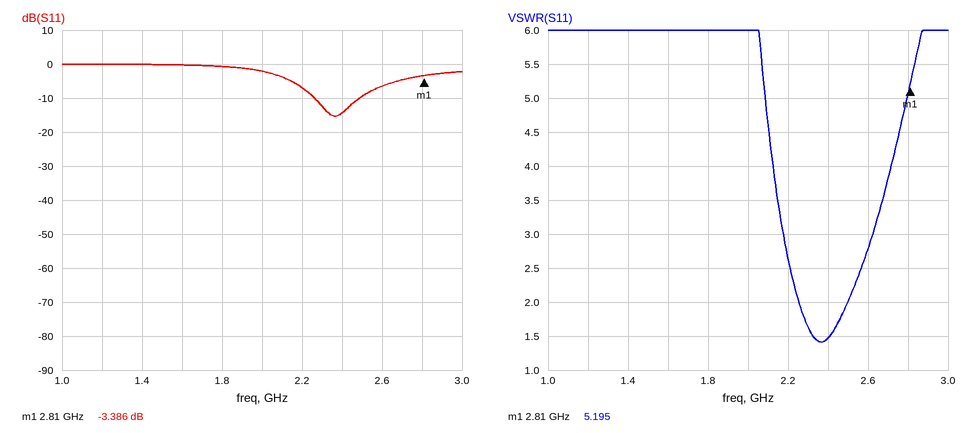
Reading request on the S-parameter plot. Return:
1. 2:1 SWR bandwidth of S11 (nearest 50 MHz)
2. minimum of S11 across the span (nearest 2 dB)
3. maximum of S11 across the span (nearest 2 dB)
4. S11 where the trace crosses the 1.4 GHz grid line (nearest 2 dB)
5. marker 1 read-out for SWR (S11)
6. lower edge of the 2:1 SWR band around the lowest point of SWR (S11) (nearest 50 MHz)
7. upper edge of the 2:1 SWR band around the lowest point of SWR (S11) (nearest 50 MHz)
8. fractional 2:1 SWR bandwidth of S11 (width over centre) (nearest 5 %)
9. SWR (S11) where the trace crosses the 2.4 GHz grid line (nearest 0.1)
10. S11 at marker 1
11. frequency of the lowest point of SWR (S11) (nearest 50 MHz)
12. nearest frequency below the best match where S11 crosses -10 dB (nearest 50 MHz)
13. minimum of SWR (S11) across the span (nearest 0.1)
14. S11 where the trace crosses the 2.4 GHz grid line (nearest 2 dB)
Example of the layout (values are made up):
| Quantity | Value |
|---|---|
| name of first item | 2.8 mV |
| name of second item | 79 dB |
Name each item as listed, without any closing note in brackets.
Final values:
| Quantity | Value |
|---|---|
| 2:1 SWR bandwidth of S11 | 250 MHz |
| minimum of S11 across the span | -16 dB |
| maximum of S11 across the span | 0 dB |
| S11 where the trace crosses the 1.4 GHz grid line | 0 dB |
| marker 1 read-out for SWR | 5.195 |
| lower edge of the 2:1 SWR band around the lowest point of SWR (S11) | 2.25 GHz |
| upper edge of the 2:1 SWR band around the lowest point of SWR (S11) | 2.50 GHz |
| fractional 2:1 SWR bandwidth of S11 (width over centre) | 10 % |
| SWR (S11) where the trace crosses the 2.4 GHz grid line | 1.5 |
| S11 at marker 1 | -3.386 dB |
| frequency of the lowest point of SWR (S11) | 2.35 GHz |
| nearest frequency below the best match where S11 crosses -10 dB | 2.25 GHz |
| minimum of SWR (S11) across the span | 1.4 |
| S11 where the trace crosses the 2.4 GHz grid line | -14 dB |
